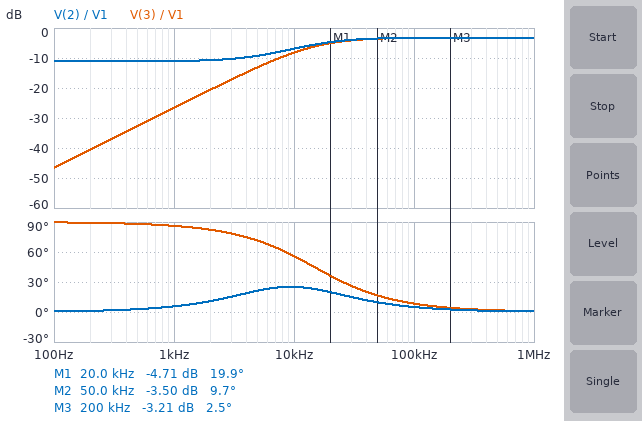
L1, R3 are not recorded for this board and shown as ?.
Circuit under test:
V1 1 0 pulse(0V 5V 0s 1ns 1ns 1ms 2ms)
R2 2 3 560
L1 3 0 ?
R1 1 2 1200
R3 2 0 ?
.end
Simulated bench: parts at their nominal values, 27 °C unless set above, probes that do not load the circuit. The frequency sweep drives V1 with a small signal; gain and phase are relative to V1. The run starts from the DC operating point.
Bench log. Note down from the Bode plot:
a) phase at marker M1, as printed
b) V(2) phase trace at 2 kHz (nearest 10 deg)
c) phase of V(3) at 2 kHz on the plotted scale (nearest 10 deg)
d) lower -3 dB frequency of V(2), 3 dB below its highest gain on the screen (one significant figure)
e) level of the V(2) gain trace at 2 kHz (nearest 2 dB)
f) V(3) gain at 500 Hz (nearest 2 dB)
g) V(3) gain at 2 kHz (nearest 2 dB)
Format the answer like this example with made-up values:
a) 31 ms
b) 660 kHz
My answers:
a) 19.9 deg
b) 10 deg
c) 80 deg
d) 10 kHz
e) -10 dB
f) -32 dB
g) -20 dB
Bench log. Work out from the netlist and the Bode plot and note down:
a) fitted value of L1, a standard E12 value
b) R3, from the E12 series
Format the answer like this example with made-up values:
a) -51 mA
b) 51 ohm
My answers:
a) 15 mH
b) 2.7 kΩ
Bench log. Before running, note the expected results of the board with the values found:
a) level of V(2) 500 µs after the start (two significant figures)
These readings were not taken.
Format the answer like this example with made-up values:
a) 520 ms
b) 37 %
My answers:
a) 1.4 V
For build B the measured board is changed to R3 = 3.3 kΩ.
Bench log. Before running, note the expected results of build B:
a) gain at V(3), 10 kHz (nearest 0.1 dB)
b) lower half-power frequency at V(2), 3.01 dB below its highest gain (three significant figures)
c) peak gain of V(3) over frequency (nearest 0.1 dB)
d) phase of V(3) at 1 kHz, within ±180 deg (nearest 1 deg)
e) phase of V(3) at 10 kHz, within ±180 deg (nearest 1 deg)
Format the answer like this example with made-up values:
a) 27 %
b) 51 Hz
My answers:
a) -7.9 dB
b) 12.8 kHz
c) -2.7 dB
d) 86 deg
e) 57 deg
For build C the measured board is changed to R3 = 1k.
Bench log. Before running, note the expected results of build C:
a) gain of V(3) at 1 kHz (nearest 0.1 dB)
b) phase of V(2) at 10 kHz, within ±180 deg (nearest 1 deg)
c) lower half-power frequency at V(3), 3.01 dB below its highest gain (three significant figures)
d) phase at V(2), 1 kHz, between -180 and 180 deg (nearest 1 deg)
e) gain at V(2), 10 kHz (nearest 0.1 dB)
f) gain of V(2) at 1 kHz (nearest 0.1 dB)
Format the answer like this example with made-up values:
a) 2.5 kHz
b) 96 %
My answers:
a) -28.3 dB
b) 19 deg
c) 11.7 kHz
d) 5 deg
e) -9.3 dB
f) -12.7 dB
